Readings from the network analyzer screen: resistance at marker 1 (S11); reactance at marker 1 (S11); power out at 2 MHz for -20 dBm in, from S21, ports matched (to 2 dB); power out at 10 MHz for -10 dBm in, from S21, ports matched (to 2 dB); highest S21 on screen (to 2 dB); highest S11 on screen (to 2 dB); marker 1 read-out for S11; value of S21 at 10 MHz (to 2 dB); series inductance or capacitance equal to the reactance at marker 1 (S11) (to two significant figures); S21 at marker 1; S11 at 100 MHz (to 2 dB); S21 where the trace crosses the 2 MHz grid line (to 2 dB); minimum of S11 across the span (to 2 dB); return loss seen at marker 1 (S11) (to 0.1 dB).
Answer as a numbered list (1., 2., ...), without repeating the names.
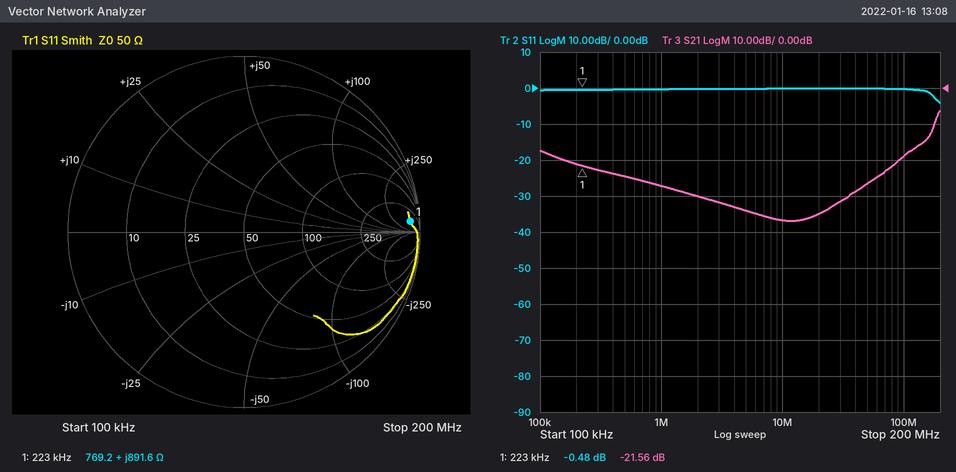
1. 769.2 Ω
2. +891.6 Ω
3. -50 dBm
4. -46 dBm
5. -6 dB
6. 0 dB
7. -0.48 dB
8. -36 dB
9. 640 µH
10. -21.56 dB
11. 0 dB
12. -30 dB
13. -4 dB
14. 0.5 dB
